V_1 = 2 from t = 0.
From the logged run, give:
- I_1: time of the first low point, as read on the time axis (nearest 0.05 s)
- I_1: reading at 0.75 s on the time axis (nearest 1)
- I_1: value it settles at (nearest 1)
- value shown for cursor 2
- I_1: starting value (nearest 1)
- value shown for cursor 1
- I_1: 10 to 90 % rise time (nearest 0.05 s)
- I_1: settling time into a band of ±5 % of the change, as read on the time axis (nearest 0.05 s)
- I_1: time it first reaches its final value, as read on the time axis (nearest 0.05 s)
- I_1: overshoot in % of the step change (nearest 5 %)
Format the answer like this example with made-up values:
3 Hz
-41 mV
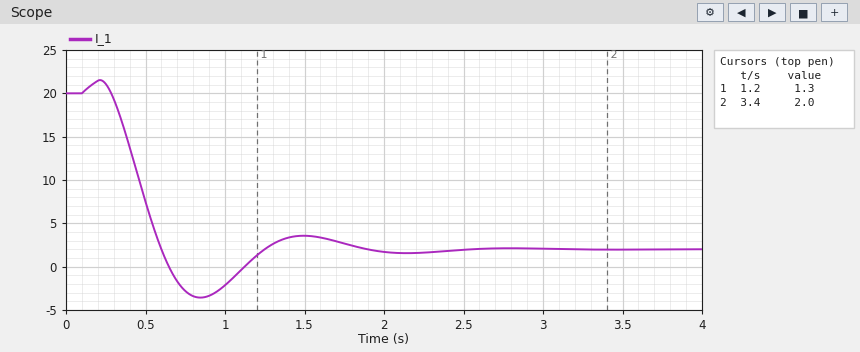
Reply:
0.85 s
-3
2
2.0
20
1.3
0.25 s
1.70 s
0.60 s
30 %
